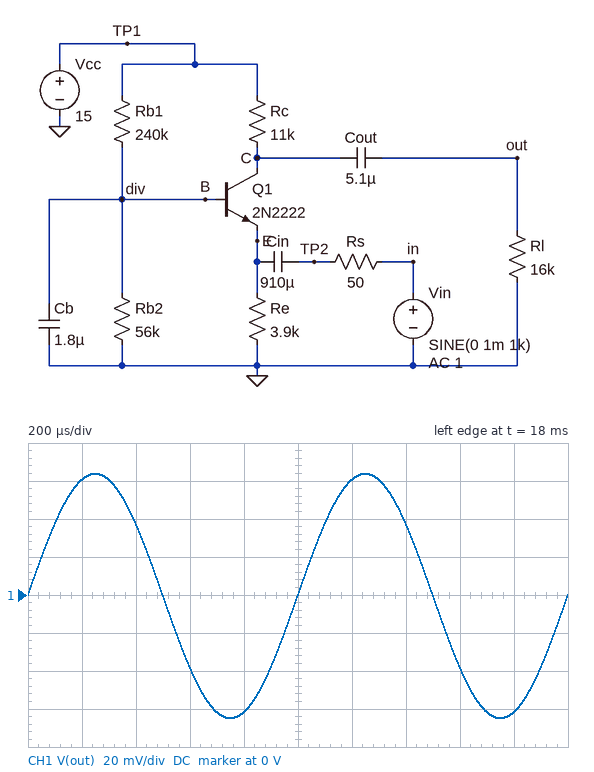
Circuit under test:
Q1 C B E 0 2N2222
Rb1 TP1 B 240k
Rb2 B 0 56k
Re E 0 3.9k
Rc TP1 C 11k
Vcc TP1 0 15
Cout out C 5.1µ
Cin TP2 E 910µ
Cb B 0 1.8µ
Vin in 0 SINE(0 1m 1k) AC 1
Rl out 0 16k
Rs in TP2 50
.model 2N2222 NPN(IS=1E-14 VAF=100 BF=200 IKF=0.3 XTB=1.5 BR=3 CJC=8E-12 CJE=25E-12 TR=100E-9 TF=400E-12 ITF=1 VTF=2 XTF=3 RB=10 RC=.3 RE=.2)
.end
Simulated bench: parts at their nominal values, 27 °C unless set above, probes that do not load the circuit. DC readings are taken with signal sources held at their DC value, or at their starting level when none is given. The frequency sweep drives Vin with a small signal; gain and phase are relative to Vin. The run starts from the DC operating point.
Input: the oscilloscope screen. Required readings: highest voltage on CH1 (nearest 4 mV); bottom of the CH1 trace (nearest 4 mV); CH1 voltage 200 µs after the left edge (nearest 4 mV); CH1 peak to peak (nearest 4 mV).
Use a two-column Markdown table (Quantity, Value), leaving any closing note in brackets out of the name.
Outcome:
| Quantity | Value |
|---|---|
| highest voltage on CH1 | 64 mV |
| bottom of the CH1 trace | -64 mV |
| CH1 voltage 200 µs after the left edge | 60 mV |
| CH1 peak to peak | 128 mV |
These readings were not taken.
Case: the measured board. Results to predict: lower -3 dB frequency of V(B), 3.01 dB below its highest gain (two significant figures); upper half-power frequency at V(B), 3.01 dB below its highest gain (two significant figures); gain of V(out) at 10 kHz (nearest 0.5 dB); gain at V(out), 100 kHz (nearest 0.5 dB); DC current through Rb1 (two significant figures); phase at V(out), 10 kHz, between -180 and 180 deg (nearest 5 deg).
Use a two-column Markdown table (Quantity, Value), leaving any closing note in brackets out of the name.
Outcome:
| Quantity | Value |
|---|---|
| lower -3 dB frequency of V(B), 3.01 dB below its highest gain | 420 mHz |
| upper half-power frequency at V(B), 3.01 dB below its highest gain | 8.4 Hz |
| gain of V(out) at 10 kHz | 36.0 dB |
| gain at V(out), 100 kHz | 36.0 dB |
| DC current through Rb1 | 51 µA |
| phase at V(out), 10 kHz, between -180 and 180 deg | 0 deg |
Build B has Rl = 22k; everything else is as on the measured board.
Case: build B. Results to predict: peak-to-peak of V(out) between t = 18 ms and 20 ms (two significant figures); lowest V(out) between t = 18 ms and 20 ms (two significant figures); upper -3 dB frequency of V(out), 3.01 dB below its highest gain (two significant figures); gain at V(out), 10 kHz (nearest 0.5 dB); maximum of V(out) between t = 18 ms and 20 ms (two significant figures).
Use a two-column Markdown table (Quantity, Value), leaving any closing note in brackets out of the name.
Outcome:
| Quantity | Value |
|---|---|
| peak-to-peak of V(out) between t = 18 ms and 20 ms | 140 mV |
| lowest V(out) between t = 18 ms and 20 ms | -73 mV |
| upper -3 dB frequency of V(out), 3.01 dB below its highest gain | 5.2 MHz |
| gain at V(out), 10 kHz | 37.0 dB |
| maximum of V(out) between t = 18 ms and 20 ms | 72 mV |
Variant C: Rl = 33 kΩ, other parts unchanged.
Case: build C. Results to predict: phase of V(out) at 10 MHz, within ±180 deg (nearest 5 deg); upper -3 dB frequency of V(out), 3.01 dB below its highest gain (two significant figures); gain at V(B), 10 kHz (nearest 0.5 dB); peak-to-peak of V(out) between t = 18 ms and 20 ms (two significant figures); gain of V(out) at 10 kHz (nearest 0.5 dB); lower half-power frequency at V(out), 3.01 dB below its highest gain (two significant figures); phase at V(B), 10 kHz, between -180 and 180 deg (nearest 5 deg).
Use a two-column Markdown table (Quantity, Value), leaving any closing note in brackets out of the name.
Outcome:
| Quantity | Value |
|---|---|
| phase of V(out) at 10 MHz, within ±180 deg | -70 deg |
| upper -3 dB frequency of V(out), 3.01 dB below its highest gain | 4.7 MHz |
| gain at V(B), 10 kHz | -66.5 dB |
| peak-to-peak of V(out) between t = 18 ms and 20 ms | 160 mV |
| gain of V(out) at 10 kHz | 38.0 dB |
| lower half-power frequency at V(out), 3.01 dB below its highest gain | 7.1 Hz |
| phase at V(B), 10 kHz, between -180 and 180 deg | -65 deg |
